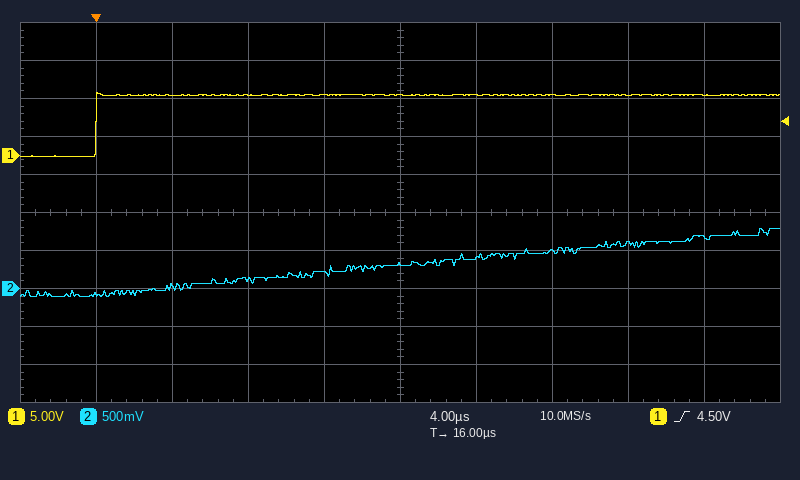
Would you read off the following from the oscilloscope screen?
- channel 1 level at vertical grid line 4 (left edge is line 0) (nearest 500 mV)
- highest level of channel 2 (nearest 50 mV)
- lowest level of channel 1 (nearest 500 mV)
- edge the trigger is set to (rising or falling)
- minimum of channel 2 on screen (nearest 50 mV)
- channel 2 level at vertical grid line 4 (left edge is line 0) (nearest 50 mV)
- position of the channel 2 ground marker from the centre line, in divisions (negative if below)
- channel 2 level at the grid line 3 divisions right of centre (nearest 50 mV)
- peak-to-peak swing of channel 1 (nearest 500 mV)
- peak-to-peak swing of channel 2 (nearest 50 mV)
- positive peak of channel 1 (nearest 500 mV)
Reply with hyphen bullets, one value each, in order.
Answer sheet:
- 8.0 V
- 800 mV
- 0.0 V
- rising
- -100 mV
- 200 mV
- -2.0 div
- 600 mV
- 8.5 V
- 900 mV
- 8.5 V
